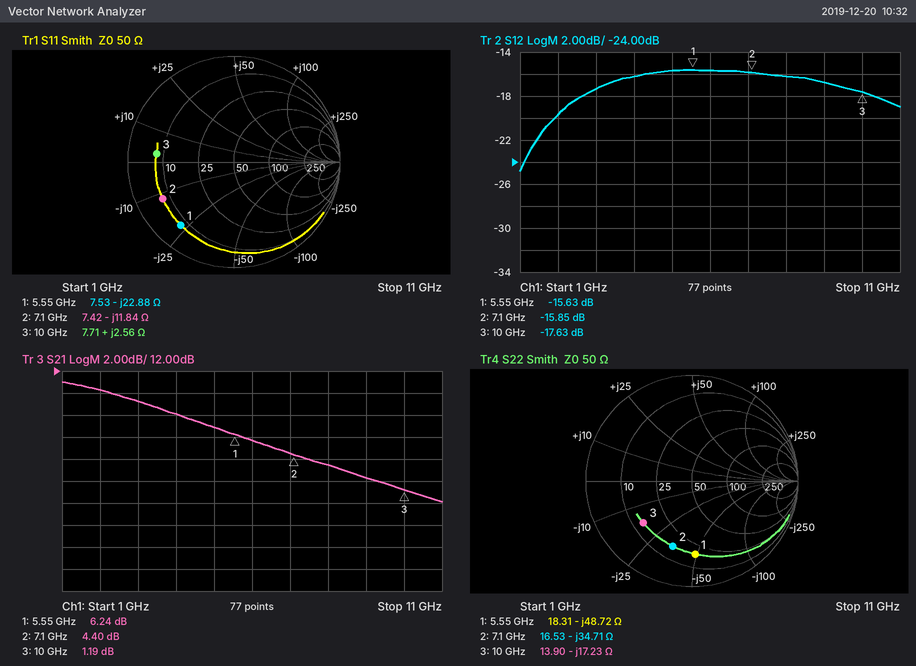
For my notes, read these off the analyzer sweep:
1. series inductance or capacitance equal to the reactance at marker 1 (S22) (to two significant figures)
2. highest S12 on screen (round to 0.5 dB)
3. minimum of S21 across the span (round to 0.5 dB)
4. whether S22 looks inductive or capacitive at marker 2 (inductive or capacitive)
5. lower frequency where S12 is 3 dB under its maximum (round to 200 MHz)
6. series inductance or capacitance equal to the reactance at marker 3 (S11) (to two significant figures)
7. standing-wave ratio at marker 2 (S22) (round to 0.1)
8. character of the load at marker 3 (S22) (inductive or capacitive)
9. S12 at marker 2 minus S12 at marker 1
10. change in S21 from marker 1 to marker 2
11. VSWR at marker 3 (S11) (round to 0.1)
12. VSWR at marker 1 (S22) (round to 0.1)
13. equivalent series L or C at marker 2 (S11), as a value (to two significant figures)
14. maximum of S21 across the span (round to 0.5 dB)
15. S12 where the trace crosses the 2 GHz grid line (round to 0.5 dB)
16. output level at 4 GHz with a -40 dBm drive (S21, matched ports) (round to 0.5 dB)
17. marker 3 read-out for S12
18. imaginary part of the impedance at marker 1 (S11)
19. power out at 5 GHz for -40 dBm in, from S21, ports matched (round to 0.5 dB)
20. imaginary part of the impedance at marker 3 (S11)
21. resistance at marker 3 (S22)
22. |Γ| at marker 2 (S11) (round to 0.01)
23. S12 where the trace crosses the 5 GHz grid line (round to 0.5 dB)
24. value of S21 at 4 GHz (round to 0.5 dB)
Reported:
590 fF
-15.5 dB
0.0 dB
capacitive
2.4 GHz
41 pH
4.6
capacitive
-0.22 dB
-1.84 dB
6.5
5.5
1.9 pF
11.0 dB
-19.5 dB
-32.0 dBm
-17.63 dB
-22.88 Ω
-33.0 dBm
+2.56 Ω
13.90 Ω
0.75
-15.5 dB
8.0 dB
